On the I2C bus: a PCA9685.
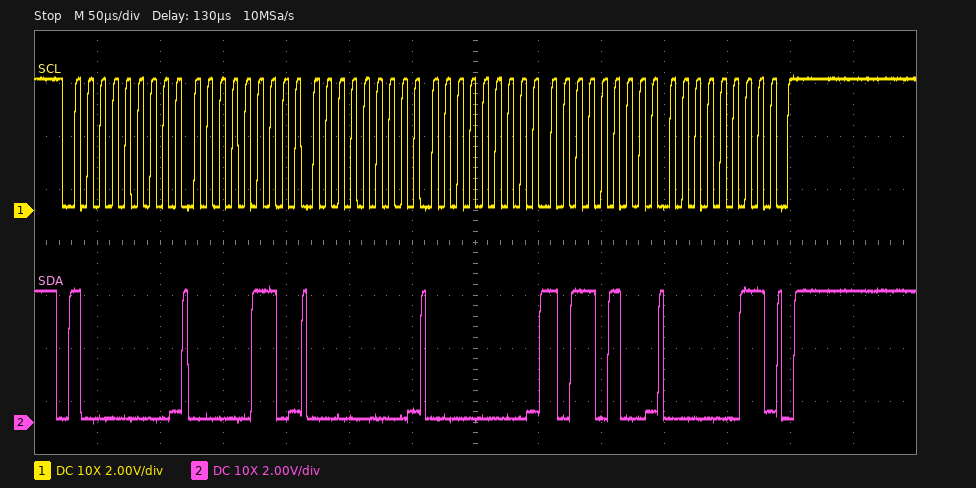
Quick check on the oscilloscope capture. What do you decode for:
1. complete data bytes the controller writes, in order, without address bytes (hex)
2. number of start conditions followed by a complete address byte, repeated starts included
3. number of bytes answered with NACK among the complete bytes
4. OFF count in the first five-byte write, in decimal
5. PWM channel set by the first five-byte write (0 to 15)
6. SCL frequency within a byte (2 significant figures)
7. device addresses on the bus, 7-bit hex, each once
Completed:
06 00 00 B4 03
1
0
948
0
100 kHz
0x40
